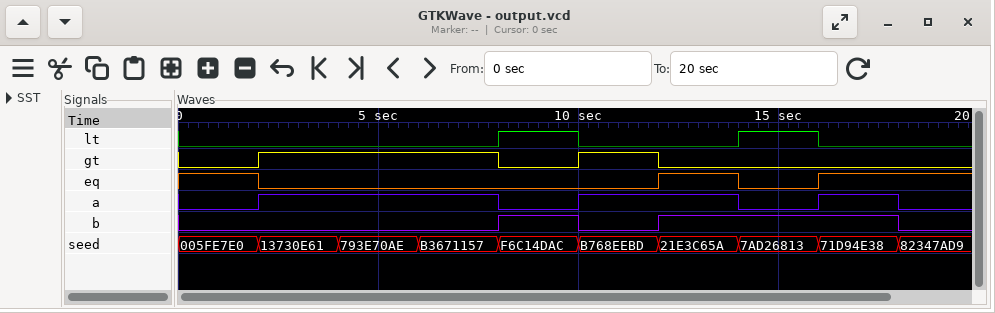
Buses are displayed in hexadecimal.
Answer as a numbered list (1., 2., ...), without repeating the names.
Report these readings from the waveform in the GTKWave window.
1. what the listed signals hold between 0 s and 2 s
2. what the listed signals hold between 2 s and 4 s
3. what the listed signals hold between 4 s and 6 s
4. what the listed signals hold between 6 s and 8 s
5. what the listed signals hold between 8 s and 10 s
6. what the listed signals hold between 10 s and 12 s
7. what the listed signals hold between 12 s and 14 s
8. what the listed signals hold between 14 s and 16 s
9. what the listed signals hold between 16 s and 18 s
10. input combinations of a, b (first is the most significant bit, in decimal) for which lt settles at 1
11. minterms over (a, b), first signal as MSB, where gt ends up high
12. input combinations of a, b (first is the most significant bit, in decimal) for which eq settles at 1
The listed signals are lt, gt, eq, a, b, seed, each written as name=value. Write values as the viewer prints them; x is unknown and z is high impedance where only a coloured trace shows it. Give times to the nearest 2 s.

1. lt=0, gt=0, eq=1, a=0, b=0, seed=005FE7E0
2. lt=0, gt=1, eq=0, a=1, b=0, seed=13730E61
3. lt=0, gt=1, eq=0, a=1, b=0, seed=793E70AE
4. lt=0, gt=1, eq=0, a=1, b=0, seed=B3671157
5. lt=1, gt=0, eq=0, a=0, b=1, seed=F6C14DAC
6. lt=0, gt=1, eq=0, a=1, b=0, seed=B768EEBD
7. lt=0, gt=0, eq=1, a=1, b=1, seed=21E3C65A
8. lt=1, gt=0, eq=0, a=0, b=1, seed=7AD26813
9. lt=0, gt=0, eq=1, a=1, b=1, seed=71D94E38
10. 1
11. 2
12. 0, 3
